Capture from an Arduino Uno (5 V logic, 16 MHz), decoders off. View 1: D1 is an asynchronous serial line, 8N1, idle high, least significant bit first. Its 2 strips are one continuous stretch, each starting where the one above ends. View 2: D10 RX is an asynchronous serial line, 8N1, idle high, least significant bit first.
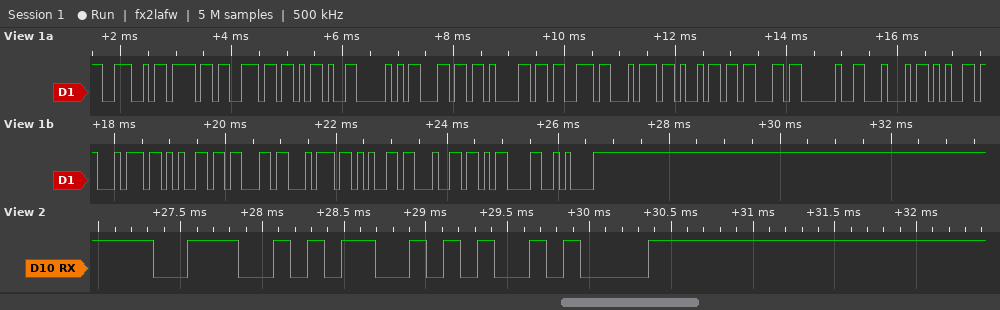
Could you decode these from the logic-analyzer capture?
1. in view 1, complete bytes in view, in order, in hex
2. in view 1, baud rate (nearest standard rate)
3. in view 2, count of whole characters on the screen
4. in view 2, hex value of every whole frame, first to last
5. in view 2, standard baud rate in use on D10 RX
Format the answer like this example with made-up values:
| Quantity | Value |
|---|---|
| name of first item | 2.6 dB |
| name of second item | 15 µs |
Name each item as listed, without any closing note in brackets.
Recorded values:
| Quantity | Value |
|---|---|
| in view 1, complete bytes in view, in order, in hex | 0x4E 0x6F 0x6E 0x2D 0x50 0x6C 0x61 0x73 0x74 0x69 0x63 0x20 0x44 0x65 0x74 0x65 0x63 0x74 0x65 0x64 0x0D 0x0A |
| in view 1, baud rate | 9600 baud |
| in view 2, count of whole characters on the screen | 3 |
| in view 2, hex value of every whole frame, first to last | 4E 53 0A |
| in view 2, standard baud rate in use on D10 RX | 9600 baud |
